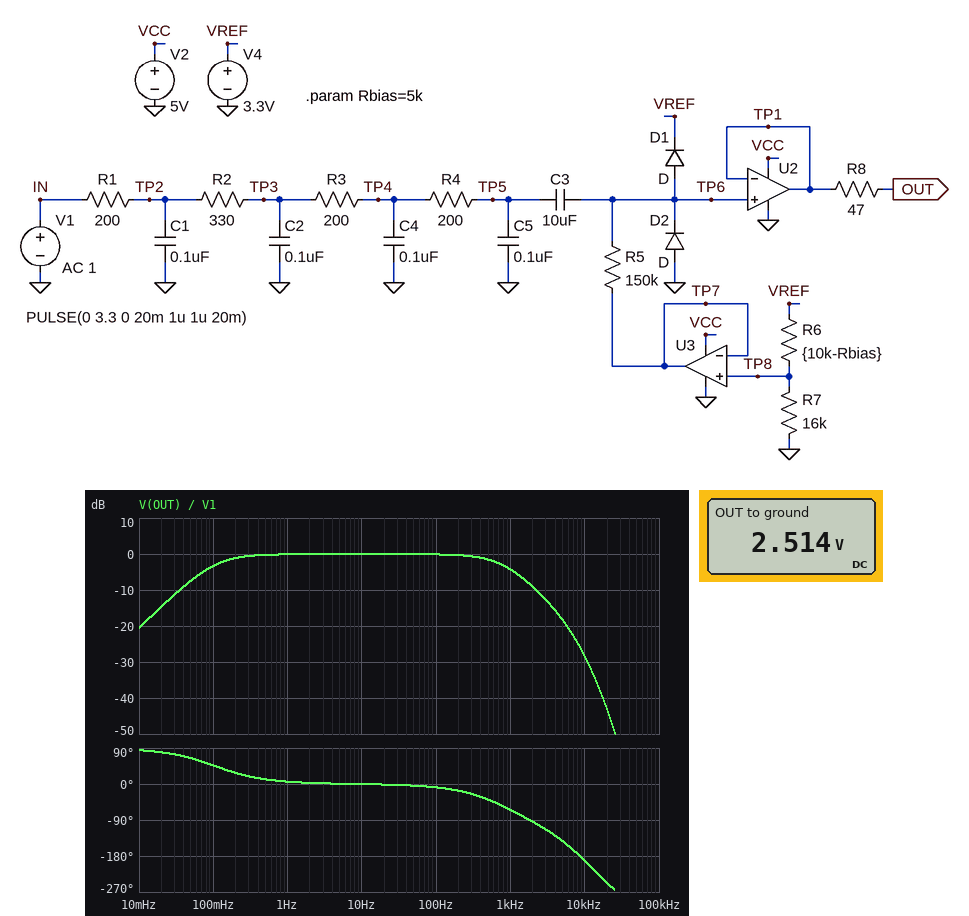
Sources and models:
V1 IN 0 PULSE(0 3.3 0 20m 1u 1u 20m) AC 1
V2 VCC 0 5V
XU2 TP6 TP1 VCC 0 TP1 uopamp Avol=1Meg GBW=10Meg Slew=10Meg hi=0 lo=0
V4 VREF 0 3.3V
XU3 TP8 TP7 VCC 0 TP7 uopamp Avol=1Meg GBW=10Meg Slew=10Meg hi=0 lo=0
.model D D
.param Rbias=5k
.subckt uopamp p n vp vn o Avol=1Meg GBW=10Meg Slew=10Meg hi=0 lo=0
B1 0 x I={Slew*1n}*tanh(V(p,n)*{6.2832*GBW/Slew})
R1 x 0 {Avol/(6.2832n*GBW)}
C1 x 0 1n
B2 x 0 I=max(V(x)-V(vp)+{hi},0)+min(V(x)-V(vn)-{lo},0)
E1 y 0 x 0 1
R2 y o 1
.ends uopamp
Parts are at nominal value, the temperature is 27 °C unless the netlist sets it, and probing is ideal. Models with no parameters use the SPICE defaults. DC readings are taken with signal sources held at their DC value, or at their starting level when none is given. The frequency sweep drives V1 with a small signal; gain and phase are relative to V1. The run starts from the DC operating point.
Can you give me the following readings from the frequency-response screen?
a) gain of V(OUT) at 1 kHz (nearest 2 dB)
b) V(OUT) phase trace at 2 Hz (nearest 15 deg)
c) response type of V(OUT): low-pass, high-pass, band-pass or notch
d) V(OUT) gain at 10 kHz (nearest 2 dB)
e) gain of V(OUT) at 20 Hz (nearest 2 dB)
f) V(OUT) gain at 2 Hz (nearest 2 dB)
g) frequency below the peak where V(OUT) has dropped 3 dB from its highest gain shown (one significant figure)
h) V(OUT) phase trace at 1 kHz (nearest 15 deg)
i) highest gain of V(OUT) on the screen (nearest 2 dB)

-4 dB
0 deg
band-pass
-28 dB
0 dB
0 dB
100 mHz
-60 deg
0 dB
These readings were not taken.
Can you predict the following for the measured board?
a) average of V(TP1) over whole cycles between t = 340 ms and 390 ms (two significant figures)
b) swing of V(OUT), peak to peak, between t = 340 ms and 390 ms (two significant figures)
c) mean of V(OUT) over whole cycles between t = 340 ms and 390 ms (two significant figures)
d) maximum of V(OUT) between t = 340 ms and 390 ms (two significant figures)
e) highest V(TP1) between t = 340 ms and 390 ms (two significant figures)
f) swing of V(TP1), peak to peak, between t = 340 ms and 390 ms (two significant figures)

2.4 V
3.0 V
2.4 V
3.9 V
3.9 V
3.0 V
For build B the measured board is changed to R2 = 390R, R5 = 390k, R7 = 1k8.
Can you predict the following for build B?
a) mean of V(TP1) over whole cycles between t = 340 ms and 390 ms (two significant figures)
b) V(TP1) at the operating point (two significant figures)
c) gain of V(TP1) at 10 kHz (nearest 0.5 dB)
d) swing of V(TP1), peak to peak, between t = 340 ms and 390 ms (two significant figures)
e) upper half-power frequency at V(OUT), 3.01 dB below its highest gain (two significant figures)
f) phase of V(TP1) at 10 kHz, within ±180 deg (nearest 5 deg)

2.3 V
870 mV
-29.5 dB
3.1 V
720 Hz
165 deg
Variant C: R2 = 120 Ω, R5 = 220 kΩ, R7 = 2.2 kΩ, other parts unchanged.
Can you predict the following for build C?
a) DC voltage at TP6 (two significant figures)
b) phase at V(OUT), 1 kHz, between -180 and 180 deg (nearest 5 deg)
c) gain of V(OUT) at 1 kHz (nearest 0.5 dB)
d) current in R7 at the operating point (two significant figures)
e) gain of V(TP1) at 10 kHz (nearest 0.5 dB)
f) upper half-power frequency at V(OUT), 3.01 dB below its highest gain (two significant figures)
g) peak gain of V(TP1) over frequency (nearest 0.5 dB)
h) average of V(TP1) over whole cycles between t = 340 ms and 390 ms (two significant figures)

1.0 V
-55 deg
-2.5 dB
460 µA
-24.5 dB
1.1 kHz
0 dB
2.2 V
